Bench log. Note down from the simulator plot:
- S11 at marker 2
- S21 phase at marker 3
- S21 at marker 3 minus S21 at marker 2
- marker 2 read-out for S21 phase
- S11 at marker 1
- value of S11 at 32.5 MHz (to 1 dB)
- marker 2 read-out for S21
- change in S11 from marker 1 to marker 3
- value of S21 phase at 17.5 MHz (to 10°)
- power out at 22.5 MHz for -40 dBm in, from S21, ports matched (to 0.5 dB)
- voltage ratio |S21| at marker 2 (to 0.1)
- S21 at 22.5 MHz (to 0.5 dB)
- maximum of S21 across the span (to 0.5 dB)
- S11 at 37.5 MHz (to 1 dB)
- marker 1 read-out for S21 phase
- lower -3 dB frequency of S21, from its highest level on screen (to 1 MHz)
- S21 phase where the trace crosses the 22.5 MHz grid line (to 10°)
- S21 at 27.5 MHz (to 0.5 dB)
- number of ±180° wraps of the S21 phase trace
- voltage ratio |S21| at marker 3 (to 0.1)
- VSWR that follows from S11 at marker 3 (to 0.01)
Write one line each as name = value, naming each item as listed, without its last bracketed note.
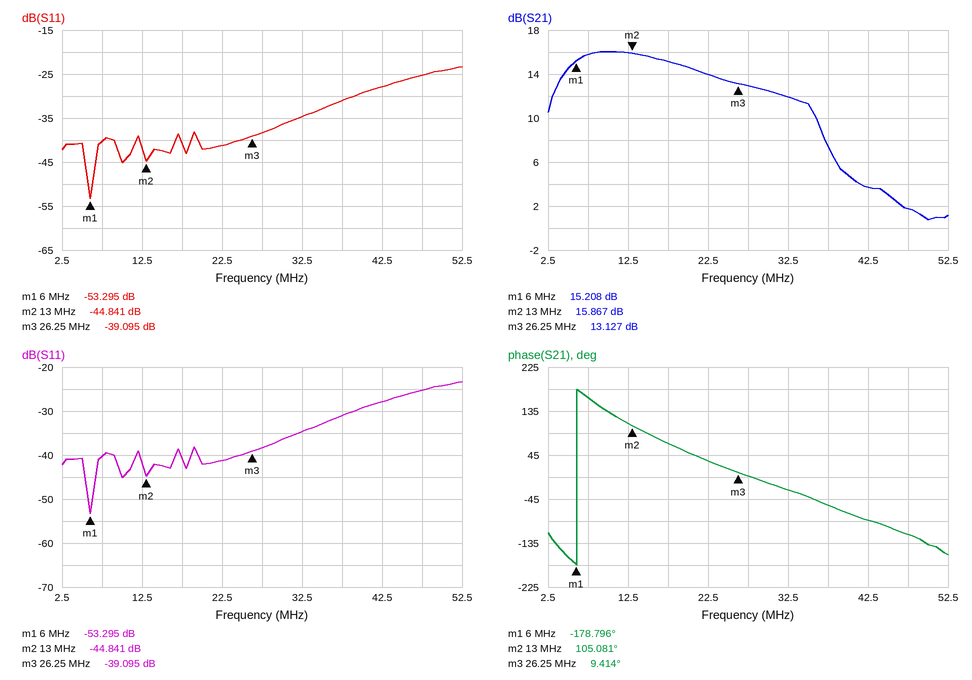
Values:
S11 at marker 2 = -44.841 dB
S21 phase at marker 3 = 9.414°
S21 at marker 3 minus S21 at marker 2 = -2.740 dB
marker 2 read-out for S21 phase = 105.081°
S11 at marker 1 = -53.295 dB
value of S11 at 32.5 MHz = -35 dB
marker 2 read-out for S21 = 15.867 dB
change in S11 from marker 1 to marker 3 = 14.200 dB
value of S21 phase at 17.5 MHz = 70°
power out at 22.5 MHz for -40 dBm in, from S21, ports matched = -26.0 dBm
voltage ratio |S21| at marker 2 = 6.2
S21 at 22.5 MHz = 14.0 dB
maximum of S21 across the span = 16.0 dB
S11 at 37.5 MHz = -31 dB
marker 1 read-out for S21 phase = -178.796°
lower -3 dB frequency of S21, from its highest level on screen = 4 MHz
S21 phase where the trace crosses the 22.5 MHz grid line = 30°
S21 at 27.5 MHz = 13.0 dB
number of ±180° wraps of the S21 phase trace = 1
voltage ratio |S21| at marker 3 = 4.5
VSWR that follows from S11 at marker 3 = 1.02
